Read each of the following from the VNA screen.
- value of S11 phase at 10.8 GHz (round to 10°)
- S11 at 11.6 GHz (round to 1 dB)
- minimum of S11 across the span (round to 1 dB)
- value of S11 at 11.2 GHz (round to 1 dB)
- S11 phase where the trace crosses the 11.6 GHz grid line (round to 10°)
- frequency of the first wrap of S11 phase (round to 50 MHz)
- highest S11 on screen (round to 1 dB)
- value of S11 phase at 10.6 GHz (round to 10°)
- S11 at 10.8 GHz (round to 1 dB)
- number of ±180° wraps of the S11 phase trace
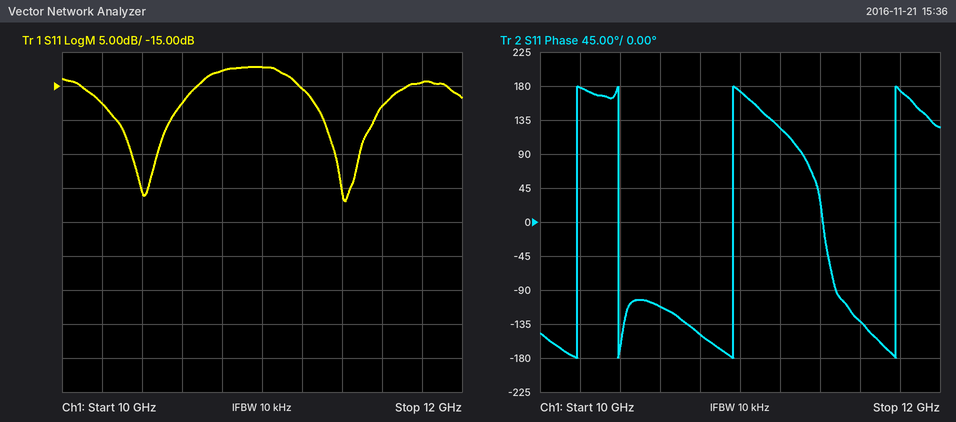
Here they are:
-150°
-18 dB
-32 dB
-15 dB
-130°
10.20 GHz
-12 dB
-110°
-13 dB
4
